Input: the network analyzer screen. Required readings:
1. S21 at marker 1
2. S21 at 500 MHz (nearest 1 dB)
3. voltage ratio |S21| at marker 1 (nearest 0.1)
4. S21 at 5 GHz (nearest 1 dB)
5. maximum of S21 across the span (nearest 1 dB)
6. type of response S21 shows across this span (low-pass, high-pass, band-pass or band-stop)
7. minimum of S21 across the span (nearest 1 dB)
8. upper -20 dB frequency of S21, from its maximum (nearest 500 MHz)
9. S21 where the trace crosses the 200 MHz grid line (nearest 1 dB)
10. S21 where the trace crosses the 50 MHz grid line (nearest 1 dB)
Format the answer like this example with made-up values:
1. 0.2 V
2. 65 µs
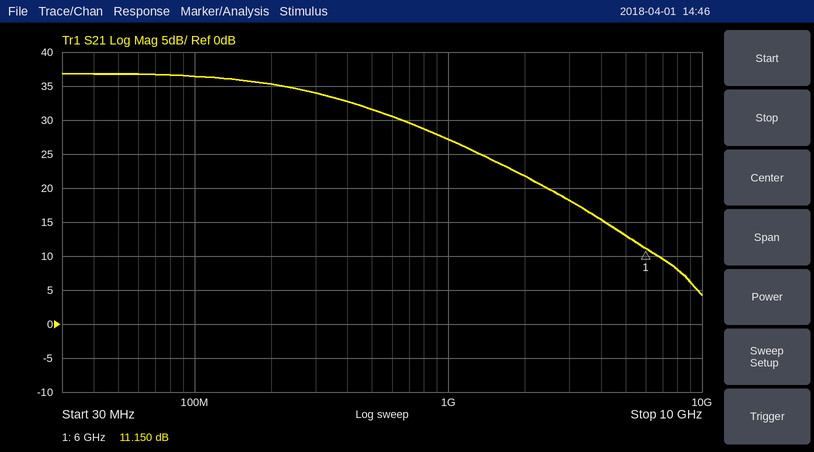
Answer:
1. 11.150 dB
2. 32 dB
3. 3.6
4. 13 dB
5. 37 dB
6. low-pass
7. 4 dB
8. 3.5 GHz
9. 35 dB
10. 37 dB
